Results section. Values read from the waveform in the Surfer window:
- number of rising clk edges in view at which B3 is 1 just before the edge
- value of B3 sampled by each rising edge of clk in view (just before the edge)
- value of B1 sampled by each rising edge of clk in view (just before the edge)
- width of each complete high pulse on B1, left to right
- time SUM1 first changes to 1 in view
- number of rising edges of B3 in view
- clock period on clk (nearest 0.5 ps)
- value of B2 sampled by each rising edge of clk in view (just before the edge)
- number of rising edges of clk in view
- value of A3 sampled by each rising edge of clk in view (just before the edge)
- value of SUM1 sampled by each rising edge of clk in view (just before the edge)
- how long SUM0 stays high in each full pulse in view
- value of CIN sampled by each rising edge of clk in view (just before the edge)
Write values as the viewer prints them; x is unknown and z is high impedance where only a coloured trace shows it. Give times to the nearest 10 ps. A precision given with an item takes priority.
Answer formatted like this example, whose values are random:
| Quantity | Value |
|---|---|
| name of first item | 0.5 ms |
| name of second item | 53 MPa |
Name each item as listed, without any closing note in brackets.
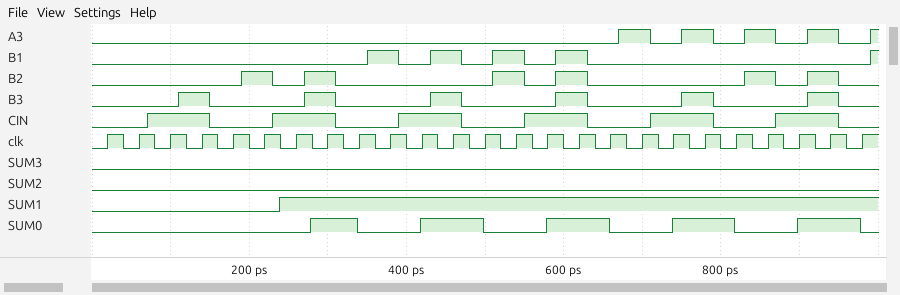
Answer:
| Quantity | Value |
|---|---|
| number of rising clk edges in view at which B3 is 1 just before the edge | 6 |
| value of B3 sampled by each rising edge of clk in view | 0 0 0 1 0 0 0 1 0 0 0 1 0 0 0 1 0 0 0 1 0 0 0 1 0 |
| value of B1 sampled by each rising edge of clk in view | 0 0 0 0 0 0 0 0 0 1 0 1 0 1 0 1 0 0 0 0 0 0 0 0 0 |
| width of each complete high pulse on B1, left to right | 40 ps, 40 ps, 40 ps, 40 ps |
| time SUM1 first changes to 1 in view | 240 ps |
| number of rising edges of B3 in view | 6 |
| clock period on clk | 40 ps |
| value of B2 sampled by each rising edge of clk in view | 0 0 0 0 0 1 0 1 0 0 0 0 0 1 0 1 0 0 0 0 0 1 0 1 0 |
| number of rising edges of clk in view | 25 |
| value of A3 sampled by each rising edge of clk in view | 0 0 0 0 0 0 0 0 0 0 0 0 0 0 0 0 0 1 0 1 0 1 0 1 0 |
| value of SUM1 sampled by each rising edge of clk in view | 0 0 0 0 0 0 1 1 1 1 1 1 1 1 1 1 1 1 1 1 1 1 1 1 1 |
| how long SUM0 stays high in each full pulse in view | 60 ps, 80 ps, 80 ps, 80 ps, 80 ps |
| value of CIN sampled by each rising edge of clk in view | 0 0 1 1 0 0 1 1 0 0 1 1 0 0 1 1 0 0 1 1 0 0 1 1 0 |
